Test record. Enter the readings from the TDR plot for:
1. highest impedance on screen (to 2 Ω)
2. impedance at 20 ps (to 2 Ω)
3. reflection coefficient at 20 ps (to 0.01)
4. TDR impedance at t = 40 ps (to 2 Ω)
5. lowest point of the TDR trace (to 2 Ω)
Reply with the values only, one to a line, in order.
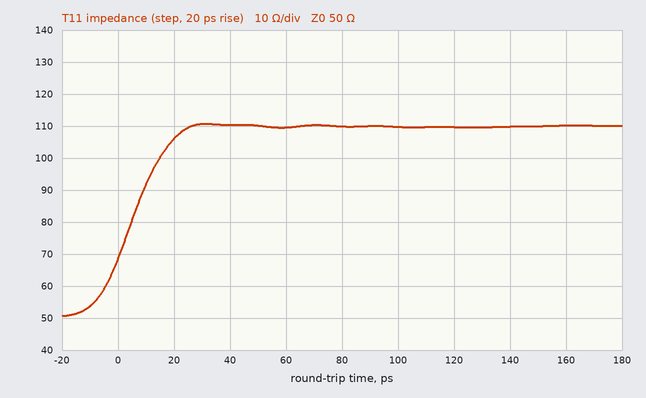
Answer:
110 Ω
106 Ω
+0.36
110 Ω
50 Ω
